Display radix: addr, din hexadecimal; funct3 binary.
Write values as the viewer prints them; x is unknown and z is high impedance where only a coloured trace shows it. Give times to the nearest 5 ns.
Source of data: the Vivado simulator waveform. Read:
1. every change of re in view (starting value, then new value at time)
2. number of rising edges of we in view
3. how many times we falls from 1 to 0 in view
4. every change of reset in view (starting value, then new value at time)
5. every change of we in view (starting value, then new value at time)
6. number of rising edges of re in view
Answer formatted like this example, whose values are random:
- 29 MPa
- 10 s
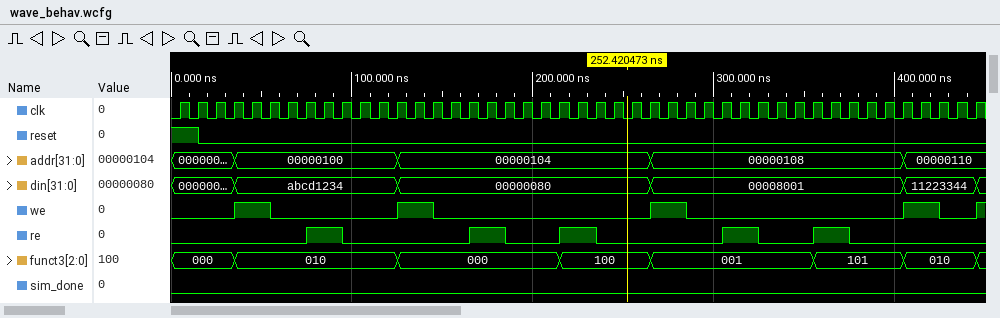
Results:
- 0, 1 at 75 ns, 0 at 95 ns, 1 at 165 ns, 0 at 185 ns, 1 at 215 ns, 0 at 235 ns, 1 at 305 ns, 0 at 325 ns, 1 at 355 ns, 0 at 375 ns
- 5
- 4
- 1, 0 at 15 ns
- 0, 1 at 35 ns, 0 at 55 ns, 1 at 125 ns, 0 at 145 ns, 1 at 265 ns, 0 at 285 ns, 1 at 405 ns, 0 at 425 ns, 1 at 445 ns
- 5
